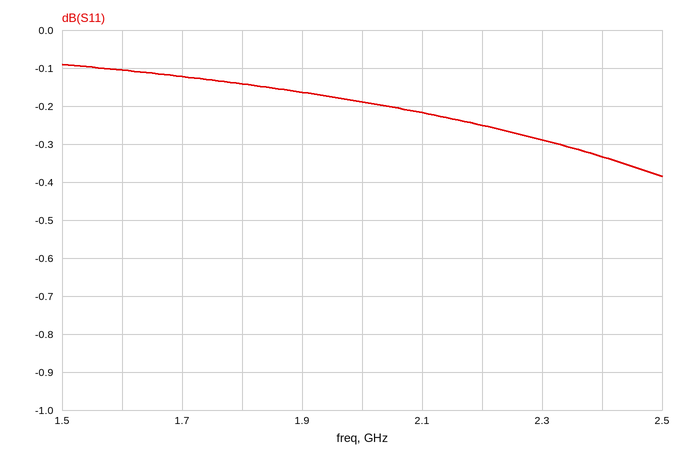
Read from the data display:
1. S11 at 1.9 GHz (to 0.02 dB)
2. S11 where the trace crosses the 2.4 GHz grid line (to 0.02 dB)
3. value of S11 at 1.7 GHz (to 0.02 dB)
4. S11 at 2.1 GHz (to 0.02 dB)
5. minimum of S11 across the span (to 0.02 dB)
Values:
-0.16 dB
-0.34 dB
-0.12 dB
-0.22 dB
-0.38 dB
